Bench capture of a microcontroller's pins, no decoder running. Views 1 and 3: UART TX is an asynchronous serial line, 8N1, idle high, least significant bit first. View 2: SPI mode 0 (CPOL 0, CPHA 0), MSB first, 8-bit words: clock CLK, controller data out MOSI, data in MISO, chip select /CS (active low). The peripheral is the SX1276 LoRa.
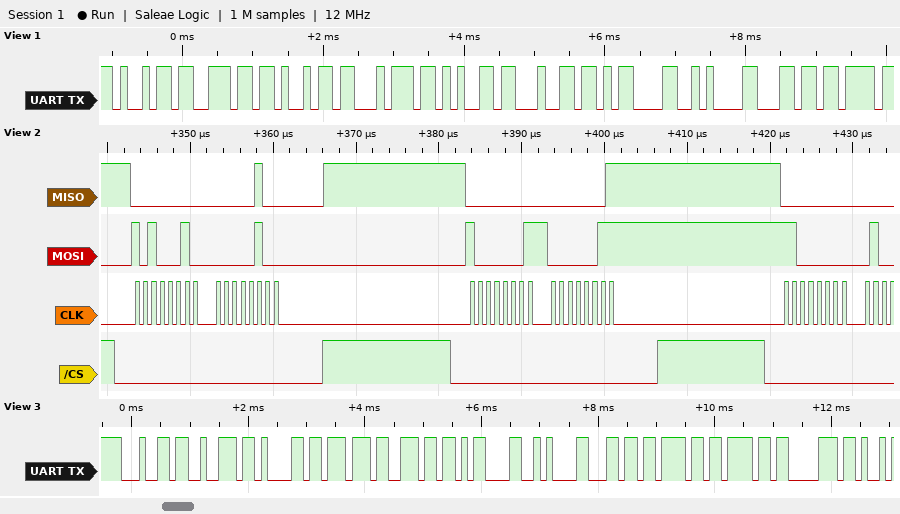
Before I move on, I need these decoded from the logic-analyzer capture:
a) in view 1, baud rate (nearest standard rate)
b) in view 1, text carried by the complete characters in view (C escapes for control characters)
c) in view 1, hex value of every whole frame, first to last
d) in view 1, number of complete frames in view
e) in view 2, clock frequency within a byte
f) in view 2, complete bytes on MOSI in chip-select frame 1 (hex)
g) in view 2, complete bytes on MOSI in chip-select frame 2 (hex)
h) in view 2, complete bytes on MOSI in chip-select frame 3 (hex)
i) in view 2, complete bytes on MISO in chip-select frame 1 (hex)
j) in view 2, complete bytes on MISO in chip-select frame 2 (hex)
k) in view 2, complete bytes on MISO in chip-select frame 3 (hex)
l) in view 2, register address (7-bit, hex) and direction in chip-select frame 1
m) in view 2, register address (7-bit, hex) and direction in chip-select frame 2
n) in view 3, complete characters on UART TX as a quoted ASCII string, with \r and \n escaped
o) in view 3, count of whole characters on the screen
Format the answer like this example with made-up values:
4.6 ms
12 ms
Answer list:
9600 baud
"inited\r\nl"
69 6E 69 74 65 64 0D 0A 6C
9
1 MHz
0xA2 0x04
0x81 0x03
0xC0
0x00 0x04
0x00 0x01
0x00
0x22 write
0x01 write
"drawn\r\nloop"
11
